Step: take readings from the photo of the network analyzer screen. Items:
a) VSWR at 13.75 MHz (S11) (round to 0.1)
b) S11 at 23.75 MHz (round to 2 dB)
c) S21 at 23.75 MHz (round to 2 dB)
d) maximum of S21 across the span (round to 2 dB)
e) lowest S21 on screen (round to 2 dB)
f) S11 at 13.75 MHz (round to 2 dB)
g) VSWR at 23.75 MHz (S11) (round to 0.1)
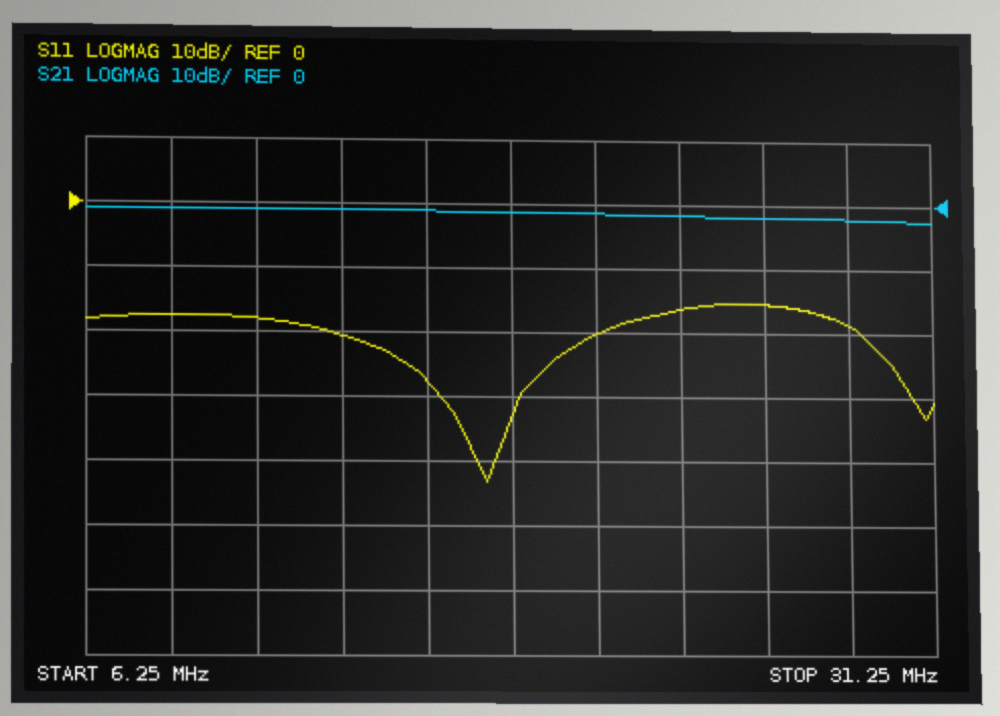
1.2
-16 dB
-2 dB
0 dB
-2 dB
-20 dB
1.4
